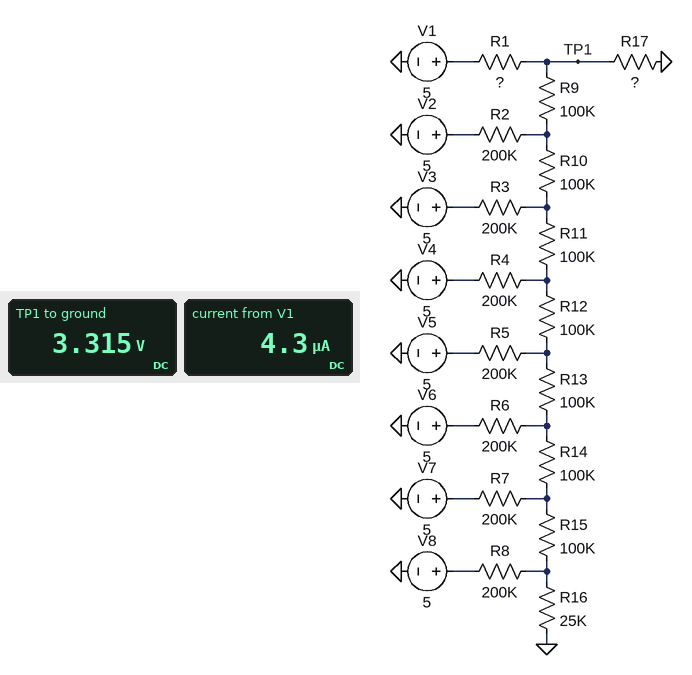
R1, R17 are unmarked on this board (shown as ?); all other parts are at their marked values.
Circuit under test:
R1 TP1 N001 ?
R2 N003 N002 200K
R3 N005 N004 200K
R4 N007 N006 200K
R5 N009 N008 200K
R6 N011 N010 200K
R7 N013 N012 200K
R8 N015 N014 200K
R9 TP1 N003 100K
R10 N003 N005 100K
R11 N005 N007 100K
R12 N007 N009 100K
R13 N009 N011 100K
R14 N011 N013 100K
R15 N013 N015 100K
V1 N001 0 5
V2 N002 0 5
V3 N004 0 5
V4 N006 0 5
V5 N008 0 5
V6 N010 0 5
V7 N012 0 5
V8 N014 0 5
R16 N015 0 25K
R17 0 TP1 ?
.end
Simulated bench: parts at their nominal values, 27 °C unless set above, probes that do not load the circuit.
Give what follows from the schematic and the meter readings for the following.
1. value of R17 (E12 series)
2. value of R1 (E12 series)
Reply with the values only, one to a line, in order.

270 kΩ
390 kΩ
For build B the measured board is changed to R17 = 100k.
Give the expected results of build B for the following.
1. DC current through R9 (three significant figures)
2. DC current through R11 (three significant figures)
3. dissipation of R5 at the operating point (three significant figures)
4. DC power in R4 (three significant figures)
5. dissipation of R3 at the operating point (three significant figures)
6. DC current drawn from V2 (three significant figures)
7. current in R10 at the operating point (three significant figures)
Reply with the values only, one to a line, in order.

13.9 µA
2.31 µA
2.28 µW
1.83 µW
3.49 µW
7.42 µA
6.48 µA
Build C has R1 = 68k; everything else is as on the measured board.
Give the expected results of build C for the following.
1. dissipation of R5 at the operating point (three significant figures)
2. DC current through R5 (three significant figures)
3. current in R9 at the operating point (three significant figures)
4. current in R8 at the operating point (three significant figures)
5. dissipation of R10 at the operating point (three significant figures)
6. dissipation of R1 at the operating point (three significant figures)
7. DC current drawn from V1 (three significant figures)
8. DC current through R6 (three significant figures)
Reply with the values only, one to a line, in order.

1.50 µW
2.74 µA
3.59 µA
20.0 µA
176 nW
9.67 µW
11.9 µA
5.12 µA
